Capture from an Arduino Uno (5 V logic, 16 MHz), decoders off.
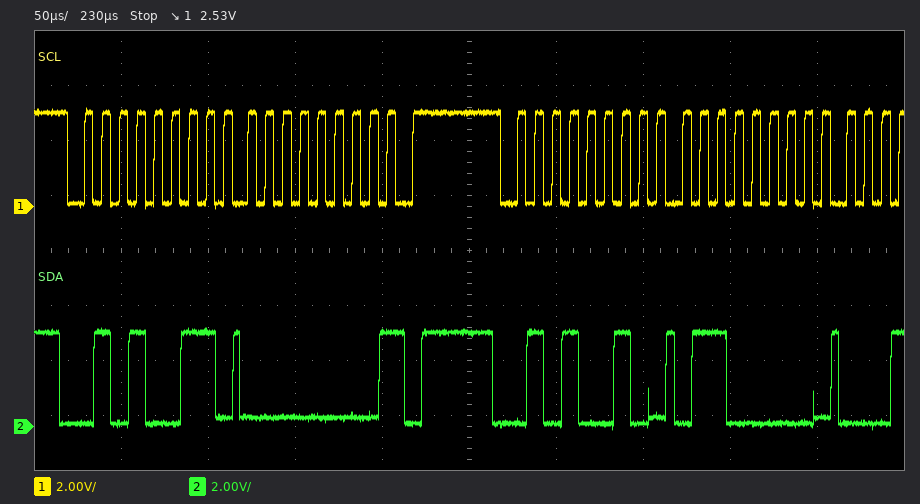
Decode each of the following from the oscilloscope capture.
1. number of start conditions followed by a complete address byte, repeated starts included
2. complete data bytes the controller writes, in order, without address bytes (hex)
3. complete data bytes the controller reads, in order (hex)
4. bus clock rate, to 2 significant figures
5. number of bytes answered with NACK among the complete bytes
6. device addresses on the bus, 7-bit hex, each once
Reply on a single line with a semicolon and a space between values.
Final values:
2; 60; 00; 100 kHz; 1; 0x29
